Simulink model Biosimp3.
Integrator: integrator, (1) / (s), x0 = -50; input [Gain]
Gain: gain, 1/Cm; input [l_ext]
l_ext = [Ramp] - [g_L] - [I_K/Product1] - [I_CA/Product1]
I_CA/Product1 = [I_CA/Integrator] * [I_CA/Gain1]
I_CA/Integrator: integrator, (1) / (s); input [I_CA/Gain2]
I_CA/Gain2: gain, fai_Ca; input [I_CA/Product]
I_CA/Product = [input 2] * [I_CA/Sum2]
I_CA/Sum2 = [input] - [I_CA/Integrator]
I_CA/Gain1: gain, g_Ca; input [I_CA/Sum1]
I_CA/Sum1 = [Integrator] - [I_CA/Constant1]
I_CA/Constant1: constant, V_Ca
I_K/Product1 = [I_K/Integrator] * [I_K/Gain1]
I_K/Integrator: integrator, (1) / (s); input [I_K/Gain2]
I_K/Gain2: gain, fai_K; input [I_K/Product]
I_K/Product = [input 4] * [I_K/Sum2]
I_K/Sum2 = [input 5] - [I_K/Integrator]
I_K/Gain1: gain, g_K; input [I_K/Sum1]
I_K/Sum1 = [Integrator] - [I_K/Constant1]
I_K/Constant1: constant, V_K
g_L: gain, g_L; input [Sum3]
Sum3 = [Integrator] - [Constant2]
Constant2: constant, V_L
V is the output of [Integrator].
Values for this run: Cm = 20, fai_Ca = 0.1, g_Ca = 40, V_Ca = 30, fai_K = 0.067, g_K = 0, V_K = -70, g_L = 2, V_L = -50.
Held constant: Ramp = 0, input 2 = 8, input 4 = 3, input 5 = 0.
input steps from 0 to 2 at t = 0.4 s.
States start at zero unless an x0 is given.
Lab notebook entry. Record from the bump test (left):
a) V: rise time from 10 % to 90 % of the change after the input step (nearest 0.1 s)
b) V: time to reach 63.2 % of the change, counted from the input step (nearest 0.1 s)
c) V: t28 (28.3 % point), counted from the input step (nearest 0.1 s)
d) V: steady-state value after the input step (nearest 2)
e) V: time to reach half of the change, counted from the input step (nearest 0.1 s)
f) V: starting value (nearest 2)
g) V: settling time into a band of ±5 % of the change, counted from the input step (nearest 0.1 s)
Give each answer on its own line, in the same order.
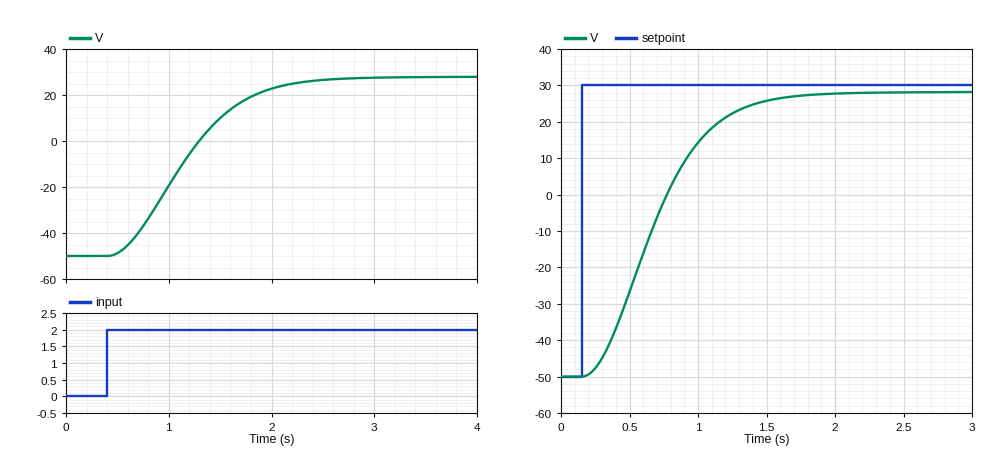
1.2 s
0.9 s
0.5 s
28
0.7 s
-50
1.7 s
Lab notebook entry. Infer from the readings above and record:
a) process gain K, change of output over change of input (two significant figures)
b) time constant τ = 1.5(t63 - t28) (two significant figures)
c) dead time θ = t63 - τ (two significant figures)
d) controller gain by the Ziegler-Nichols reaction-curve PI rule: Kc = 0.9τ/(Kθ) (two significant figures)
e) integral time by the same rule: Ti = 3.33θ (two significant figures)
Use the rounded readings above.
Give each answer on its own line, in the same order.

39
0.60 s
0.30 s
0.046
1.00 s
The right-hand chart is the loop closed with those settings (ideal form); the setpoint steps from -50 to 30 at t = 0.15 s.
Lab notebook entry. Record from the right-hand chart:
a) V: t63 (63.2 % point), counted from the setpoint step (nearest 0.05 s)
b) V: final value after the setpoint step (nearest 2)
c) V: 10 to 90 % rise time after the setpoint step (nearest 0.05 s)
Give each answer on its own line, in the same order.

0.60 s
28
0.85 s
